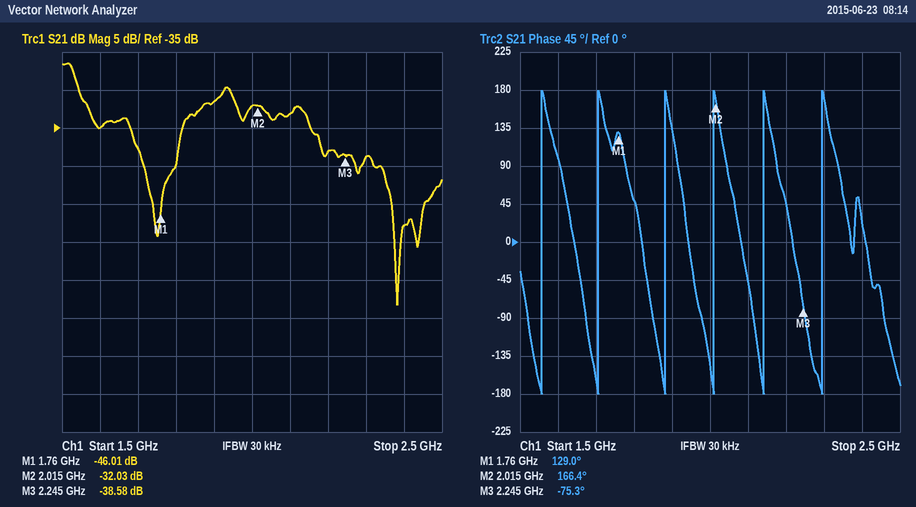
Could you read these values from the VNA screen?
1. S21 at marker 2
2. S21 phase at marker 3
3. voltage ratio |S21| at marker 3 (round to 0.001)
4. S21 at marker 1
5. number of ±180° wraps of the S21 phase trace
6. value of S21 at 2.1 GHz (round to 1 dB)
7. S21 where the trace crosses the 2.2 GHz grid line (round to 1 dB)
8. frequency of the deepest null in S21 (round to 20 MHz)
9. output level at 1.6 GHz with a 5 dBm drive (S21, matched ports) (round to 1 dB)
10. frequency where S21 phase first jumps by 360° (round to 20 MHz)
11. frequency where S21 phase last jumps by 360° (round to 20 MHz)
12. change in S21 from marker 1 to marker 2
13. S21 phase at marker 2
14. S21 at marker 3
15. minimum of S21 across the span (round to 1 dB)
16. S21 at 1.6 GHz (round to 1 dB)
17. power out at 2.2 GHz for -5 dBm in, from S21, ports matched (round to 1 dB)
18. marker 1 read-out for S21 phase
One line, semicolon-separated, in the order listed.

-32.03 dB; -75.3°; 0.012; -46.01 dB; 6; -33 dB; -38 dB; 2.38 GHz; -30 dBm; 1.56 GHz; 2.30 GHz; 13.98 dB; 166.4°; -38.58 dB; -58 dB; -35 dB; -43 dBm; 129.0°
